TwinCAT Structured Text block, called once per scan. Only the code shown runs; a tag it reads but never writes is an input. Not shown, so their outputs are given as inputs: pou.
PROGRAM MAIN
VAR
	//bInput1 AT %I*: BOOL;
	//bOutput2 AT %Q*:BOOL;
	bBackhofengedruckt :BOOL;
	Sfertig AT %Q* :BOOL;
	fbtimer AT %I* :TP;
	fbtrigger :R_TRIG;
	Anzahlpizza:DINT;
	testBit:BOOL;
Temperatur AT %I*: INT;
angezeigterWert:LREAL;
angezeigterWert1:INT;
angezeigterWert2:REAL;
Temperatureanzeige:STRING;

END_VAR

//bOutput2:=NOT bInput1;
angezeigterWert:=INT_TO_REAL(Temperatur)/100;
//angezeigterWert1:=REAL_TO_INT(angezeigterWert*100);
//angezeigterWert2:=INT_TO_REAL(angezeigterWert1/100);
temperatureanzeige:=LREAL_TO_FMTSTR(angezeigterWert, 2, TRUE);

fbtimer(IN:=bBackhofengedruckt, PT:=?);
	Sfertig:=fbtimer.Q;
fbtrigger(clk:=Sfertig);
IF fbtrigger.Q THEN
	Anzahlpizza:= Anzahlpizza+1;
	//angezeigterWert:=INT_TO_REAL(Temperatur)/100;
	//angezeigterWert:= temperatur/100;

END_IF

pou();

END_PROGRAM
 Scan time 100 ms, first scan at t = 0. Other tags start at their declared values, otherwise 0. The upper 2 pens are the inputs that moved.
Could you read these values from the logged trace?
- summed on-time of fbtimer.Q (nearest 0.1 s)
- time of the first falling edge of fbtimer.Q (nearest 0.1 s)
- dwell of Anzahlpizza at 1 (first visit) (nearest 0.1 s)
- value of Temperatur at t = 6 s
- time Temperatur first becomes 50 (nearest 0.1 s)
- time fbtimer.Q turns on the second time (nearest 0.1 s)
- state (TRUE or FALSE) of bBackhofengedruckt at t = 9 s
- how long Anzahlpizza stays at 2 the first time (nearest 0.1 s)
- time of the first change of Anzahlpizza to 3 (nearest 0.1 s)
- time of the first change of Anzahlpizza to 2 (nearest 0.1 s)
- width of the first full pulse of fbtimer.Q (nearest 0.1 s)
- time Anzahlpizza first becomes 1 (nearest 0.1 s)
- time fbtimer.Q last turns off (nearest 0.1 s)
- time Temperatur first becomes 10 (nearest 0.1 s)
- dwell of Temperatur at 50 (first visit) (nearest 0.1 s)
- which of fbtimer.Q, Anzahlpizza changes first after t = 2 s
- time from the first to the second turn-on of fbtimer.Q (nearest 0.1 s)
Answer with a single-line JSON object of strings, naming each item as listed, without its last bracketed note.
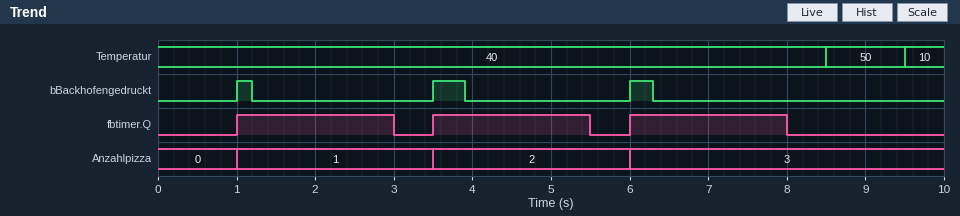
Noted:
{"summed on-time of fbtimer.Q": "6.0 s", "time of the first falling edge of fbtimer.Q": "3.0 s", "dwell of Anzahlpizza at 1 (first visit)": "2.5 s", "value of Temperatur at t = 6 s": "40", "time Temperatur first becomes 50": "8.5 s", "time fbtimer.Q turns on the second time": "3.5 s", "state (TRUE or FALSE) of bBackhofengedruckt at t = 9 s": "FALSE", "how long Anzahlpizza stays at 2 the first time": "2.5 s", "time of the first change of Anzahlpizza to 3": "6.0 s", "time of the first change of Anzahlpizza to 2": "3.5 s", "width of the first full pulse of fbtimer.Q": "2.0 s", "time Anzahlpizza first becomes 1": "1.0 s", "time fbtimer.Q last turns off": "8.0 s", "time Temperatur first becomes 10": "9.5 s", "dwell of Temperatur at 50 (first visit)": "1.0 s", "which of fbtimer.Q, Anzahlpizza changes first after t = 2 s": "fbtimer.Q", "time from the first to the second turn-on of fbtimer.Q": "2.5 s"}
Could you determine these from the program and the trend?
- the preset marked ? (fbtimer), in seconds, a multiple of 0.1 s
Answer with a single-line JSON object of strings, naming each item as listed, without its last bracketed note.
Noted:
{"the preset marked ? (fbtimer), in seconds, a multiple of 0.1 s": "2.0 s"}
